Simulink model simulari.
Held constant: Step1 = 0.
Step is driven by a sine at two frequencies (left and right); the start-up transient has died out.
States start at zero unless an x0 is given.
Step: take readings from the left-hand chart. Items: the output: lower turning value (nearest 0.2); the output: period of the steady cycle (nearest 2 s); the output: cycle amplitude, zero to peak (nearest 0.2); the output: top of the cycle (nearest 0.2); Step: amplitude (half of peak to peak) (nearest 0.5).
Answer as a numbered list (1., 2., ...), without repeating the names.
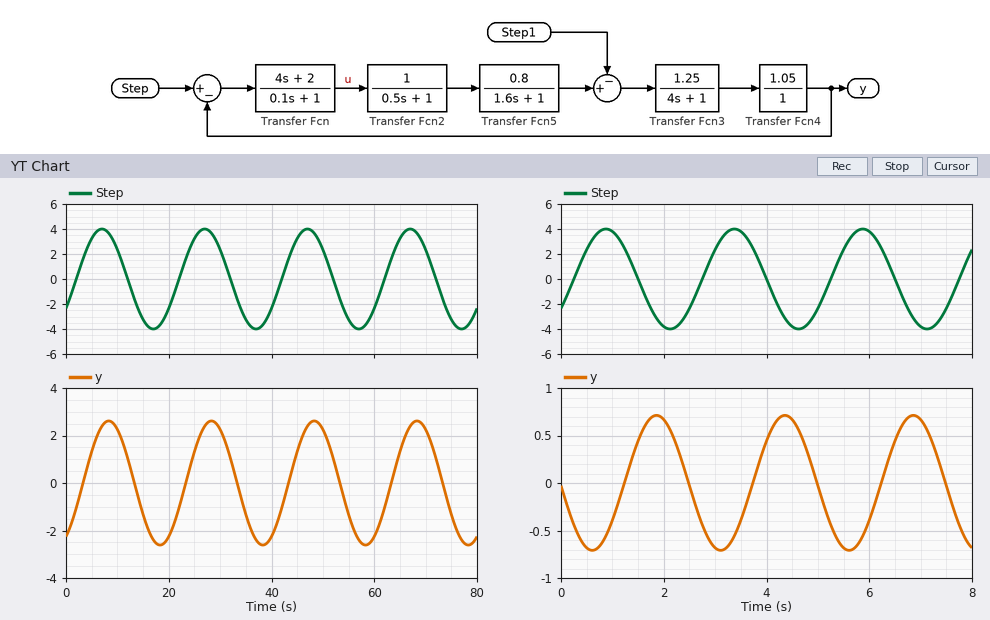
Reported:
1. -2.6
2. 20 s
3. 2.6
4. 2.6
5. 4.0
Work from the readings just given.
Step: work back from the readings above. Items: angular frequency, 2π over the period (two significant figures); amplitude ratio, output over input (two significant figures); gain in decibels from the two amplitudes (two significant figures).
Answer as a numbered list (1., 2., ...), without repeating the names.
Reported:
1. 0.31 rad/s
2. 0.65
3. -3.7 dB
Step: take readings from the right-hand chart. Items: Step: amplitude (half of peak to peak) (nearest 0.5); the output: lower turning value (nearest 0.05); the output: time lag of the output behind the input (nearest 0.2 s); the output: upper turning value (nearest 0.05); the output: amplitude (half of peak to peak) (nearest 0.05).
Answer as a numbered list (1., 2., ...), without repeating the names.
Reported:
1. 4.0
2. -0.70
3. 1.0 s
4. 0.70
5. 0.70
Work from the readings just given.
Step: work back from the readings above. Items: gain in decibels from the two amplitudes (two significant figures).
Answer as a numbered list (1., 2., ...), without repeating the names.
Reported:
1. -15 dB
